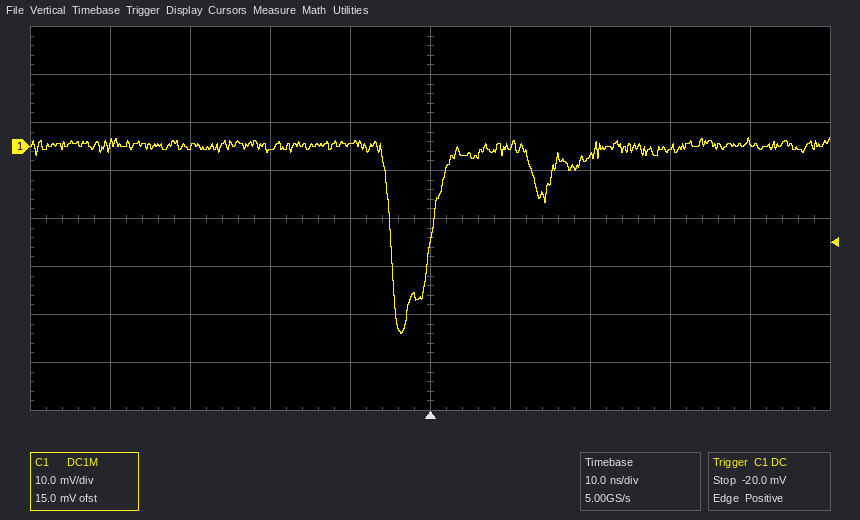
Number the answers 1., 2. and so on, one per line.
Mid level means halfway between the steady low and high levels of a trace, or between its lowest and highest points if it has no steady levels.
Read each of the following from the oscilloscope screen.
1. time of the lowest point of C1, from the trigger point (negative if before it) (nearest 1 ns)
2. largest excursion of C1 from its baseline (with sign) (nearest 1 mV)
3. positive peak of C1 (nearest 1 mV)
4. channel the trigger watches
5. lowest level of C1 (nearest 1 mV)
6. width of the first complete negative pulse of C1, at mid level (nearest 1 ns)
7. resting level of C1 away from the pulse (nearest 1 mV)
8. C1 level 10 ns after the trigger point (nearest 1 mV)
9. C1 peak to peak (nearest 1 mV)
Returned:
1. -4 ns
2. -39 mV
3. 2 mV
4. C1
5. -39 mV
6. 5 ns
7. 0 mV
8. 0 mV
9. 41 mV
